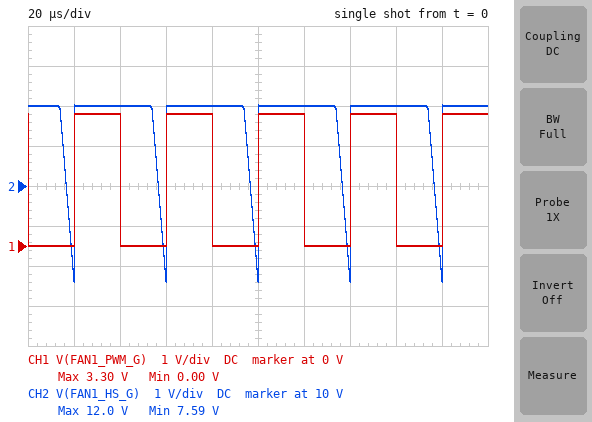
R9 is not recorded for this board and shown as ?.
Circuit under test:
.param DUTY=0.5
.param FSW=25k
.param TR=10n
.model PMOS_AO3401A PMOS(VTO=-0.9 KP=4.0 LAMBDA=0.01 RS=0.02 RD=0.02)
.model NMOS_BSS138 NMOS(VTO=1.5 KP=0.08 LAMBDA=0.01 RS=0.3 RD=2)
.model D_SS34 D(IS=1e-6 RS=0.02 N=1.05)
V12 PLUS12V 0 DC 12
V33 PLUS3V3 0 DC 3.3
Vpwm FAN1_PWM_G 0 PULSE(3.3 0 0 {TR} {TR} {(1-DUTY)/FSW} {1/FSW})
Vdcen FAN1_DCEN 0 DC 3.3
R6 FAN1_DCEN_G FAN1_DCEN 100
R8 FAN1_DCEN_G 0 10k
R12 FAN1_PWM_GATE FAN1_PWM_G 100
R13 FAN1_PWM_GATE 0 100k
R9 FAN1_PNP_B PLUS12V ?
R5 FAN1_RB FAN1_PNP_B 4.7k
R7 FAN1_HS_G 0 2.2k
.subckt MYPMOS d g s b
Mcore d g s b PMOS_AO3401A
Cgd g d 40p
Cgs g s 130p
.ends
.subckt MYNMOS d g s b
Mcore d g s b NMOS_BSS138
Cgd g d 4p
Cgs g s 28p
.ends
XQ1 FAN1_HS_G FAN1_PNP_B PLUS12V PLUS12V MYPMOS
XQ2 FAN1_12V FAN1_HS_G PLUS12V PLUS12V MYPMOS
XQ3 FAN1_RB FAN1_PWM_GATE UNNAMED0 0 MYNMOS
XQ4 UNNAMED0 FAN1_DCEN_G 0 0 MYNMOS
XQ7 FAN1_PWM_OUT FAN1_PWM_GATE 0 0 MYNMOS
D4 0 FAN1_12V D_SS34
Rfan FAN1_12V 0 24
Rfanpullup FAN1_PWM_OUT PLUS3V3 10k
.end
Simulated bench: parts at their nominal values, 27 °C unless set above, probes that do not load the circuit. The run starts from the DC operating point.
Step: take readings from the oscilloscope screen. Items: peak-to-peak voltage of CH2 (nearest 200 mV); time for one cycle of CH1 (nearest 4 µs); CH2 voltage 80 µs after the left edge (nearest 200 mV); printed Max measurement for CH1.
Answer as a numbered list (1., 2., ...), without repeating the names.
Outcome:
1. 4.4 V
2. 40 µs
3. 12.0 V
4. 3.30 V
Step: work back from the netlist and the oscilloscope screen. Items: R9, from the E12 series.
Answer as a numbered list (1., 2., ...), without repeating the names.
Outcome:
1. 33 kΩ
